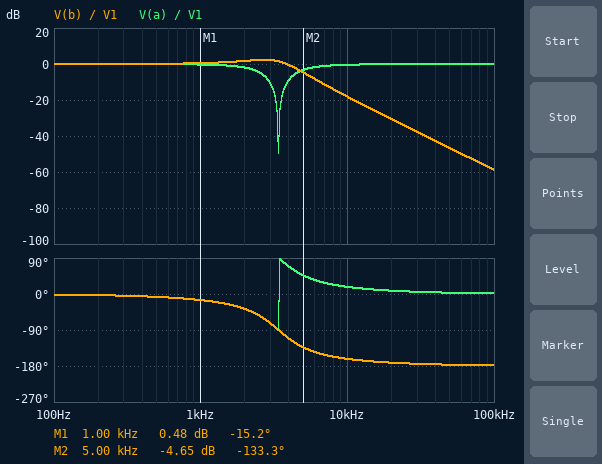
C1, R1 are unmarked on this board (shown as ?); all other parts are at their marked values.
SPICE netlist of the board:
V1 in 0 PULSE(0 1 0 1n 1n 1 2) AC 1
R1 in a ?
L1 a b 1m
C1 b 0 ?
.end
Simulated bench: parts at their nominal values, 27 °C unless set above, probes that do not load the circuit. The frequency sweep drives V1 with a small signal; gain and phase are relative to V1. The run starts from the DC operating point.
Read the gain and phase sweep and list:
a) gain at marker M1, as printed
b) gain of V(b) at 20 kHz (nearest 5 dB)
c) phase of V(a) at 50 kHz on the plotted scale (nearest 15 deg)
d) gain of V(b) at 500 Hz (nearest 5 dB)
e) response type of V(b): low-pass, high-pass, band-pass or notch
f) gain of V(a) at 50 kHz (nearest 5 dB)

0.48 dB
-30 dB
0 deg
0 dB
low-pass
0 dB
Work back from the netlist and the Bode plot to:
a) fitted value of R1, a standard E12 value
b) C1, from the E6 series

18 Ω
2.2 µF
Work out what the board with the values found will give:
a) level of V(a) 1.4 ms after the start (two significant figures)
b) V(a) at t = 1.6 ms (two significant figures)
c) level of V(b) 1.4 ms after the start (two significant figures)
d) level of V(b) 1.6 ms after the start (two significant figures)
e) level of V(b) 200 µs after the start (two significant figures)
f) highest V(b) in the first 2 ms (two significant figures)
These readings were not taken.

1.0 V
1.0 V
1.0 V
1.0 V
1.2 V
1.2 V
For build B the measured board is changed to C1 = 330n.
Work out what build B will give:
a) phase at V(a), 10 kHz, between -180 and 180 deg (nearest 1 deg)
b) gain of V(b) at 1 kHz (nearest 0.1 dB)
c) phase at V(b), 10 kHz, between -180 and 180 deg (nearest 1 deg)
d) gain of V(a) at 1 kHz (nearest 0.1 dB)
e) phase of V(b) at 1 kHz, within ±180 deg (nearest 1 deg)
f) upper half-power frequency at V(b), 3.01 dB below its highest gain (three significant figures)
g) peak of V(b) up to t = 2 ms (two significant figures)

51 deg
0.1 dB
-129 deg
0 dB
-2 deg
9.87 kHz
1.6 V
